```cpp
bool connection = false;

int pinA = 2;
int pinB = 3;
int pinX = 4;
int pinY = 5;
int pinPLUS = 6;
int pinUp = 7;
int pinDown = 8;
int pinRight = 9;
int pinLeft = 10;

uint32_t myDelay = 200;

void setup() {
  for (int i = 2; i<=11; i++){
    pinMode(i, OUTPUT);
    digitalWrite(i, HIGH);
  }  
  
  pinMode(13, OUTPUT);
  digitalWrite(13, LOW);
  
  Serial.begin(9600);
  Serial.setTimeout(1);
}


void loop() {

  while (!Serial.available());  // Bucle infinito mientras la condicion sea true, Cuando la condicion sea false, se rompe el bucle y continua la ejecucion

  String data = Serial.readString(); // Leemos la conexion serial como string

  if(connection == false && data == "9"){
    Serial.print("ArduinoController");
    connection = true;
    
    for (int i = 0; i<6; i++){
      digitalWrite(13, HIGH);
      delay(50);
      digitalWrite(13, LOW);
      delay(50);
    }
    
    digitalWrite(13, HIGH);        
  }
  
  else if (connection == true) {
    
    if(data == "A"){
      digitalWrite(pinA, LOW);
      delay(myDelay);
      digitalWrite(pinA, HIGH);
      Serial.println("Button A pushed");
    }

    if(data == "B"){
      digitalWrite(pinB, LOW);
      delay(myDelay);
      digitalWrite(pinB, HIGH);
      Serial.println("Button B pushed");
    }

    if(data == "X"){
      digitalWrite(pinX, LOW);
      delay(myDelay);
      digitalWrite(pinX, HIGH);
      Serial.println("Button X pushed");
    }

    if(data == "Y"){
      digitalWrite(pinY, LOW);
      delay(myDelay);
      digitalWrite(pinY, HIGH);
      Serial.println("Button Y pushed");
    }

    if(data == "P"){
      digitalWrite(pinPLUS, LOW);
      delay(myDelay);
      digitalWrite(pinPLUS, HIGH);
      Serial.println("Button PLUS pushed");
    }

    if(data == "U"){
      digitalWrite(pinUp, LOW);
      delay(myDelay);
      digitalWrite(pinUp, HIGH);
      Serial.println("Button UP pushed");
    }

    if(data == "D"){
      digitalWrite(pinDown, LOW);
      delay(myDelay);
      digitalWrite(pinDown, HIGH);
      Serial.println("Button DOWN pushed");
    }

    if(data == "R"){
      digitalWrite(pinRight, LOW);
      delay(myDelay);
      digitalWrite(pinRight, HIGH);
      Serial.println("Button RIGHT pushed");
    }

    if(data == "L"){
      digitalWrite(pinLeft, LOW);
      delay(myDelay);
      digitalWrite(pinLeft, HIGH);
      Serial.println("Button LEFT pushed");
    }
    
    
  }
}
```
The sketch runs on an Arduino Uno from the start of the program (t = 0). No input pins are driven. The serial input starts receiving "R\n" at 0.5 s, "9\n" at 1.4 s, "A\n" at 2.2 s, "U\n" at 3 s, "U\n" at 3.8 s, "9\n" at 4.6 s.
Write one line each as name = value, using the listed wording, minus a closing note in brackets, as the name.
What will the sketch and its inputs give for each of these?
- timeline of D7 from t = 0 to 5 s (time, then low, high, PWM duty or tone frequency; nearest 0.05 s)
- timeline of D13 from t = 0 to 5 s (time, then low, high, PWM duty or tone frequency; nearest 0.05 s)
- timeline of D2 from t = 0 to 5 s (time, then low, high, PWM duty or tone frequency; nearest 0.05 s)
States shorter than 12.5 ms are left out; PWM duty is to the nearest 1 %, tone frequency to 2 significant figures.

timeline of D7 from t = 0 to 5 s = 0 s high; 3 s low; 3.2 s high; 3.8 s low; 4 s high
timeline of D13 from t = 0 to 5 s = 0 s low; 1.4 s high; 1.45 s low; 1.5 s high; 1.55 s low; 1.6 s high; 1.65 s low; 1.7 s high; 1.75 s low; 1.8 s high; 1.85 s low; 1.9 s high; 1.95 s low; 2 s high
timeline of D2 from t = 0 to 5 s = 0 s high; 2.2 s low; 2.4 s high
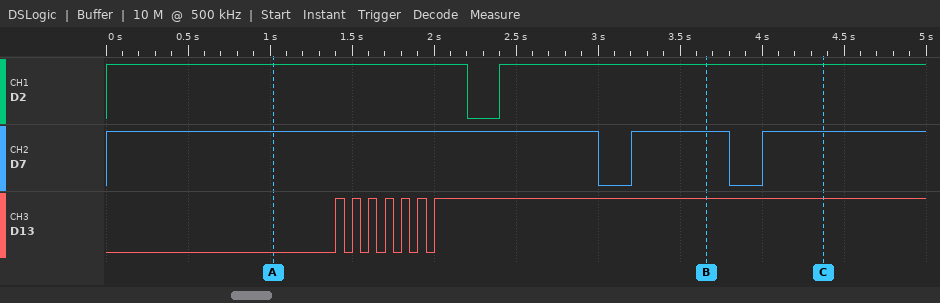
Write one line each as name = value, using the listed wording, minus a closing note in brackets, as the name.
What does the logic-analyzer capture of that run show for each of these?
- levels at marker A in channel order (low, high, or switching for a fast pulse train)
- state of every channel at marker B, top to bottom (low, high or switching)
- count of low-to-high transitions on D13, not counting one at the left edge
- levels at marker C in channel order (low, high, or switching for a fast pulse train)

levels at marker A in channel order = D2 high, D7 high, D13 low
state of every channel at marker B, top to bottom = D2 high, D7 high, D13 high
count of low-to-high transitions on D13, not counting one at the left edge = 7
levels at marker C in channel order = D2 high, D7 high, D13 high
